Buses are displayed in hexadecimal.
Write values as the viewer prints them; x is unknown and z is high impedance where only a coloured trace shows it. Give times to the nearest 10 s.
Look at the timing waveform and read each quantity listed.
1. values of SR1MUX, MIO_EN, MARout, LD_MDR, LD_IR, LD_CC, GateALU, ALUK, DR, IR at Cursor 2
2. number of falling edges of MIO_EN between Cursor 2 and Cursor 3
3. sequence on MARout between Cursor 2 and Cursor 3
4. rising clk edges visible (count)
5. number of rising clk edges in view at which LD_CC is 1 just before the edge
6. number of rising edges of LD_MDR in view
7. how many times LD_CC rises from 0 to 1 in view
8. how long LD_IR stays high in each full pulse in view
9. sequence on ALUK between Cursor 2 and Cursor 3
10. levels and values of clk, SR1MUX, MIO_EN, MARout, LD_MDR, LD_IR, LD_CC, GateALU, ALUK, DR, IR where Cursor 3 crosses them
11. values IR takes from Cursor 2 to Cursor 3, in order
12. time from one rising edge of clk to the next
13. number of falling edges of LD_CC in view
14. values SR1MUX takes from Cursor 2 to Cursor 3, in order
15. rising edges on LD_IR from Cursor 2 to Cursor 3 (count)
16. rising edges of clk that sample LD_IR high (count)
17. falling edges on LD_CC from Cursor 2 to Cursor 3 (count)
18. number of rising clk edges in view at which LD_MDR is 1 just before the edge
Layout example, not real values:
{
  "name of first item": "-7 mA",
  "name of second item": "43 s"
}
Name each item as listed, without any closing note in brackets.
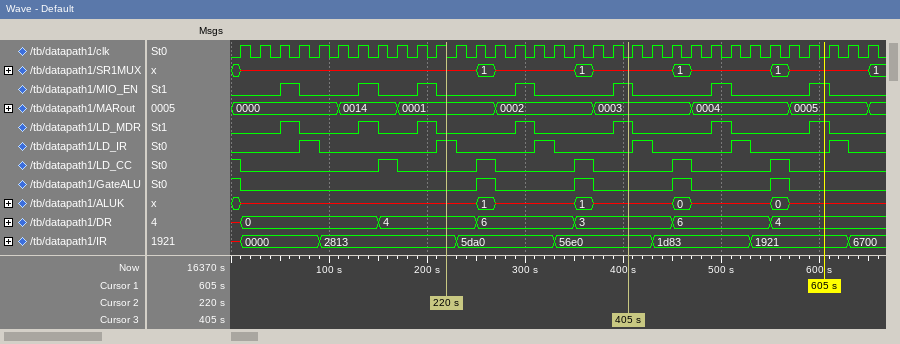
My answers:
{
  "values of SR1MUX, MIO_EN, MARout, LD_MDR, LD_IR, LD_CC, GateALU, ALUK, DR, IR at Cursor 2": "SR1MUX=x, MIO_EN=0, MARout=0001, LD_MDR=0, LD_IR=1, LD_CC=0, GateALU=0, ALUK=x, DR=4, IR=2813",
  "number of falling edges of MIO_EN between Cursor 2 and Cursor 3": "1",
  "sequence on MARout between Cursor 2 and Cursor 3": "0001, 0002, 0003",
  "rising clk edges visible": "33",
  "number of rising clk edges in view at which LD_CC is 1 just before the edge": "6",
  "number of rising edges of LD_MDR in view": "7",
  "how many times LD_CC rises from 0 to 1 in view": "5",
  "how long LD_IR stays high in each full pulse in view": "20 s, 20 s, 20 s, 20 s, 20 s, 20 s",
  "sequence on ALUK between Cursor 2 and Cursor 3": "x, 1, x, 1, x",
  "levels and values of clk, SR1MUX, MIO_EN, MARout, LD_MDR, LD_IR, LD_CC, GateALU, ALUK, DR, IR where Cursor 3 crosses them": "clk=0, SR1MUX=x, MIO_EN=1, MARout=0003, LD_MDR=1, LD_IR=0, LD_CC=0, GateALU=0, ALUK=x, DR=3, IR=56e0",
  "values IR takes from Cursor 2 to Cursor 3, in order": "2813, 5da0, 56e0",
  "time from one rising edge of clk to the next": "20 s",
  "number of falling edges of LD_CC in view": "6",
  "values SR1MUX takes from Cursor 2 to Cursor 3, in order": "x, 1, x, 1, x",
  "rising edges on LD_IR from Cursor 2 to Cursor 3": "1",
  "rising edges of clk that sample LD_IR high": "6",
  "falling edges on LD_CC from Cursor 2 to Cursor 3": "2",
  "number of rising clk edges in view at which LD_MDR is 1 just before the edge": "7"
}
